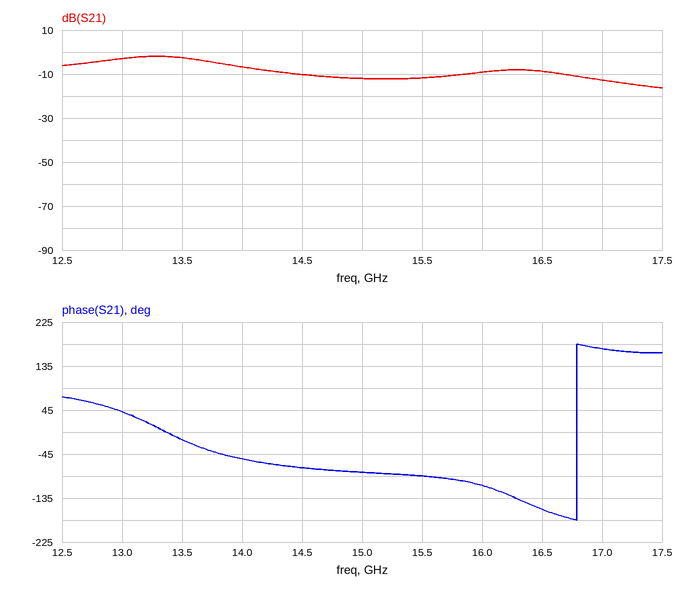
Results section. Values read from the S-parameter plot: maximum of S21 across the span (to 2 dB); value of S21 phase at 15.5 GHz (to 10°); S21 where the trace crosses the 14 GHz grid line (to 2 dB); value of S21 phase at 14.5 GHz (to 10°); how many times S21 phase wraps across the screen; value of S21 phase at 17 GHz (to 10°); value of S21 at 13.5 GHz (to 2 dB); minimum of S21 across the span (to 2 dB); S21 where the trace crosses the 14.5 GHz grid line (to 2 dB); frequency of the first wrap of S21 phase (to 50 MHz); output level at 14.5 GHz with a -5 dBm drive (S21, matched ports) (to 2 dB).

-2 dB
-90°
-6 dB
-70°
1
170°
-2 dB
-16 dB
-10 dB
16.80 GHz
-16 dBm
